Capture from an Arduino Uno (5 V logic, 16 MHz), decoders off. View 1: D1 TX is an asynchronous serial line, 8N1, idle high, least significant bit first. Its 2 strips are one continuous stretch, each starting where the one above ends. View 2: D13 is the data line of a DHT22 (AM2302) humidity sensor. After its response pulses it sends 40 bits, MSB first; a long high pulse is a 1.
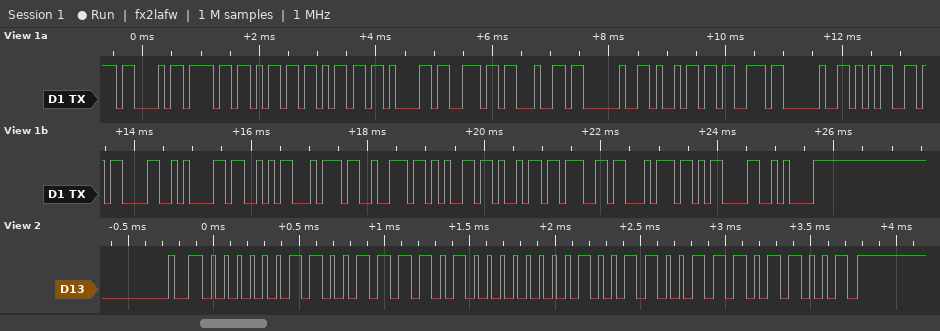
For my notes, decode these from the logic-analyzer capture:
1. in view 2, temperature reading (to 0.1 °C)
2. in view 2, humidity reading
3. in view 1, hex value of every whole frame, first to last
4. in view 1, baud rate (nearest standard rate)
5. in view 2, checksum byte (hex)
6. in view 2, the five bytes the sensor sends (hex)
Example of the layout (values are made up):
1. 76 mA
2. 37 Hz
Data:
1. 15.3 °C
2. 82.9 %
3. 43 6F 6D 6D 61 6E 64 20 69 73 20 35 0D 0A 53 74 72 65 69 67 74 0D 0A
4. 9600 baud
5. 0xD9
6. 03 3D 00 99 D9
